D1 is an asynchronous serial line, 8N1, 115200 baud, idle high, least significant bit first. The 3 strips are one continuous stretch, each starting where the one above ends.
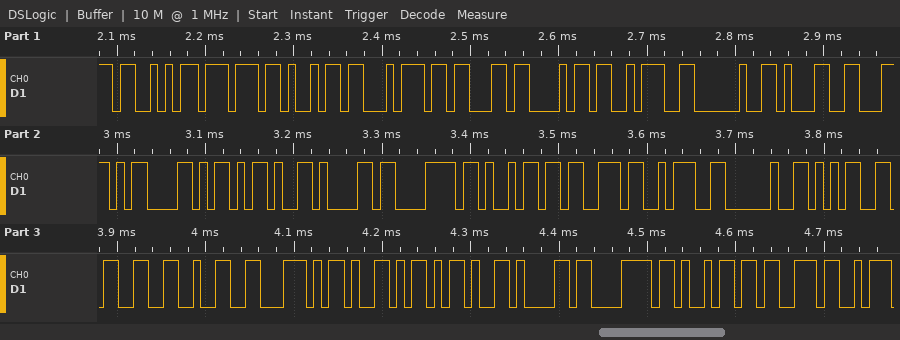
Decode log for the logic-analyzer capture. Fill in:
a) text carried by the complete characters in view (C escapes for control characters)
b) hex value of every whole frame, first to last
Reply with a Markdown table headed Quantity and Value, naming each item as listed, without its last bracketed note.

| Quantity | Value |
|---|---|
| text carried by the complete characters in view | "Switch: 1\\X-axis: 532\\Y-axis" |
| hex value of every whole frame, first to last | 0x53 0x77 0x69 0x74 0x63 0x68 0x3A 0x20 0x31 0x5C 0x58 0x2D 0x61 0x78 0x69 0x73 0x3A 0x20 0x35 0x33 0x32 0x5C 0x59 0x2D 0x61 0x78 0x69 0x73 |
